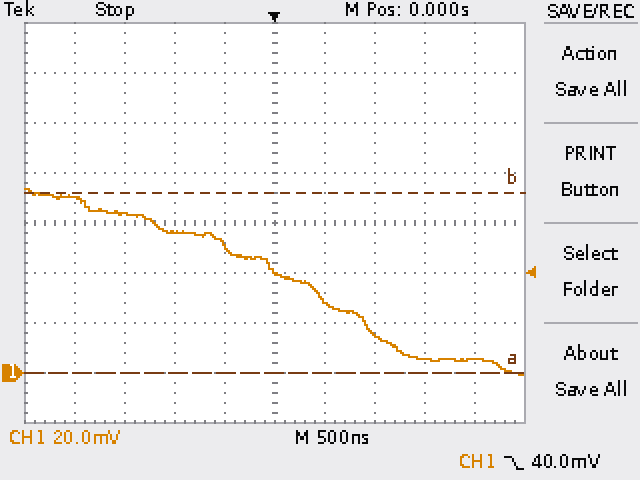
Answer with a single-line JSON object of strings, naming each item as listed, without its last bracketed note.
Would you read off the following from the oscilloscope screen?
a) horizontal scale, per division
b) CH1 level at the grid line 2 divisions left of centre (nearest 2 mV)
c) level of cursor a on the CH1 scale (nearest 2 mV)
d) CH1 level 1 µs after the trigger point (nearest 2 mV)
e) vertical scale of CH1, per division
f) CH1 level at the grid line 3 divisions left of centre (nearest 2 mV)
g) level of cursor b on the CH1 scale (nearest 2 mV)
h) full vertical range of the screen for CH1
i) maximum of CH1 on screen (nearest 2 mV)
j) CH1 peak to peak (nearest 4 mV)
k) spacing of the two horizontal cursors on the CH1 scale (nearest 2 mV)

{"horizontal scale, per division": "500 ns", "CH1 level at the grid line 2 divisions left of centre": "56 mV", "level of cursor a on the CH1 scale": "0 mV", "CH1 level 1 µs after the trigger point": "16 mV", "vertical scale of CH1, per division": "20 mV", "CH1 level at the grid line 3 divisions left of centre": "64 mV", "level of cursor b on the CH1 scale": "72 mV", "full vertical range of the screen for CH1": "160 mV", "maximum of CH1 on screen": "74 mV", "CH1 peak to peak": "76 mV", "spacing of the two horizontal cursors on the CH1 scale": "72 mV"}
